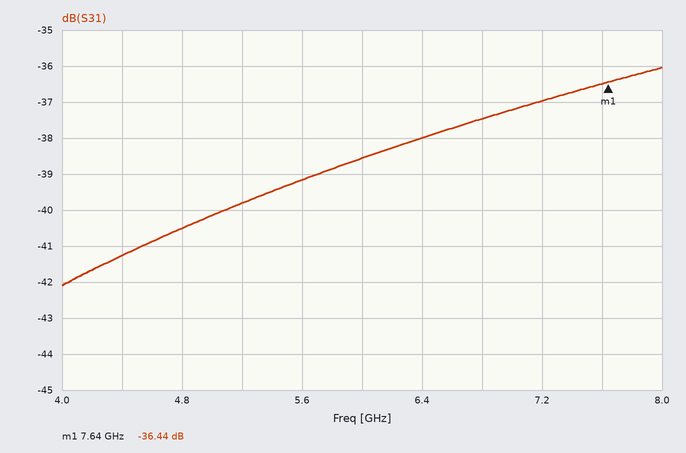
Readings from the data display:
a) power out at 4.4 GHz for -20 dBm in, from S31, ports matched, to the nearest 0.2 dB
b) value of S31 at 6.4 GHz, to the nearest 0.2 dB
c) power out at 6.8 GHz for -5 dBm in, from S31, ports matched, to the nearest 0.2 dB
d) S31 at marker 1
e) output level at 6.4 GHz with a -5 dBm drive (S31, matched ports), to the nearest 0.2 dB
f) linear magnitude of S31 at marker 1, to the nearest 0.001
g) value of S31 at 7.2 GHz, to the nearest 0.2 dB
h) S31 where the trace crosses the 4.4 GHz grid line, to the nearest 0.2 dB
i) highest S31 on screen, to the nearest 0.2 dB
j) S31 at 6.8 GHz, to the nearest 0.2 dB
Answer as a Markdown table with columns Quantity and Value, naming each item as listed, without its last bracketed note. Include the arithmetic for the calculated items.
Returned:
| Quantity | Value |
|---|---|
| power out at 4.4 GHz for -20 dBm in, from S31, ports matched, to the nearest 0.2 dB | -20 dBm + (-41.2 dB) = -61.2 dBm |
| value of S31 at 6.4 GHz, to the nearest 0.2 dB | -38.0 dB |
| power out at 6.8 GHz for -5 dBm in, from S31, ports matched, to the nearest 0.2 dB | -5 dBm + (-37.4 dB) = -42.4 dBm |
| S31 at marker 1 | -36.44 dB |
| output level at 6.4 GHz with a -5 dBm drive (S31, matched ports), to the nearest 0.2 dB | -5 dBm + (-38.0 dB) = -43.0 dBm |
| linear magnitude of S31 at marker 1, to the nearest 0.001 | 10^(-36.44/20) ≈ 0.015 |
| value of S31 at 7.2 GHz, to the nearest 0.2 dB | -37.0 dB |
| S31 where the trace crosses the 4.4 GHz grid line, to the nearest 0.2 dB | -41.2 dB |
| highest S31 on screen, to the nearest 0.2 dB | -36.0 dB |
| S31 at 6.8 GHz, to the nearest 0.2 dB | -37.4 dB |
